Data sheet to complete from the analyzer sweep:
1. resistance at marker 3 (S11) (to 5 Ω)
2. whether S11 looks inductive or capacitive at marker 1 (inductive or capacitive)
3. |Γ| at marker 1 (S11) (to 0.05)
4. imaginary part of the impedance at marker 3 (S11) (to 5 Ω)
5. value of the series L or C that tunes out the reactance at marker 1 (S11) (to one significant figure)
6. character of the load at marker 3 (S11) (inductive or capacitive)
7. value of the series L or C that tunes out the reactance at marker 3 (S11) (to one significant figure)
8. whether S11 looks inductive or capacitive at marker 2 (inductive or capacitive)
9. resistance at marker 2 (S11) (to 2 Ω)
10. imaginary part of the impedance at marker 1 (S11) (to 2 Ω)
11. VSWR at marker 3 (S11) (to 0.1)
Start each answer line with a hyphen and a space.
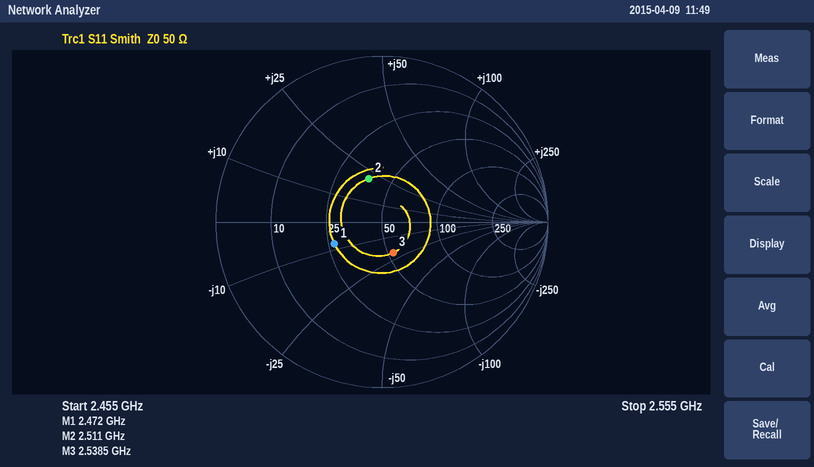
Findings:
- 55 Ω
- capacitive
- 0.30
- -20 Ω
- 500 pH
- capacitive
- 1 nH
- inductive
- 38 Ω
- -8 Ω
- 1.5
